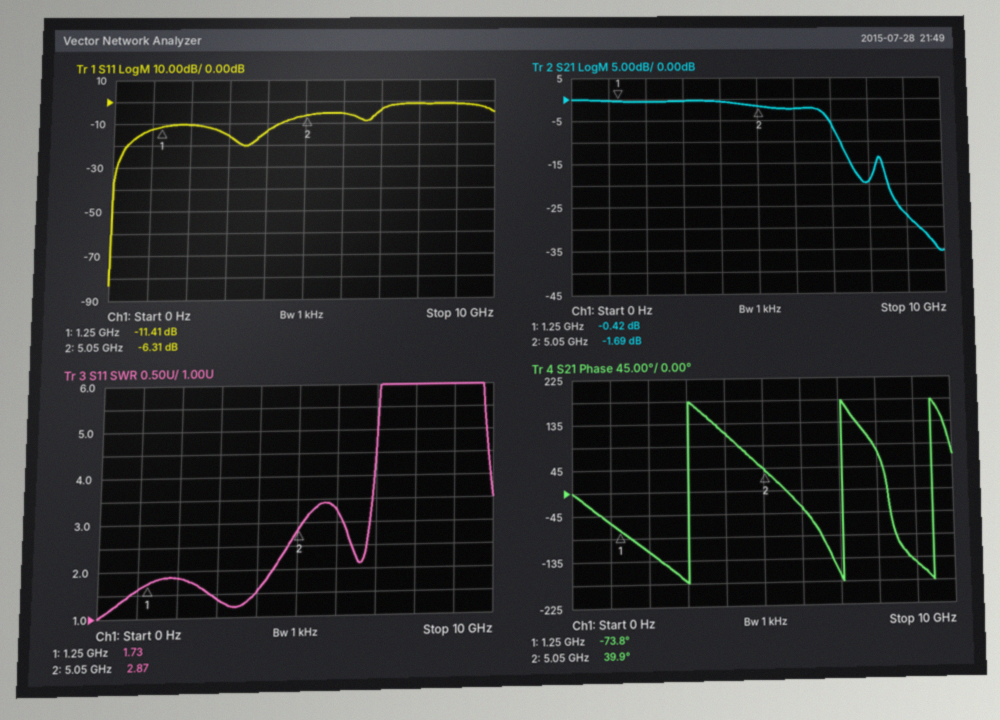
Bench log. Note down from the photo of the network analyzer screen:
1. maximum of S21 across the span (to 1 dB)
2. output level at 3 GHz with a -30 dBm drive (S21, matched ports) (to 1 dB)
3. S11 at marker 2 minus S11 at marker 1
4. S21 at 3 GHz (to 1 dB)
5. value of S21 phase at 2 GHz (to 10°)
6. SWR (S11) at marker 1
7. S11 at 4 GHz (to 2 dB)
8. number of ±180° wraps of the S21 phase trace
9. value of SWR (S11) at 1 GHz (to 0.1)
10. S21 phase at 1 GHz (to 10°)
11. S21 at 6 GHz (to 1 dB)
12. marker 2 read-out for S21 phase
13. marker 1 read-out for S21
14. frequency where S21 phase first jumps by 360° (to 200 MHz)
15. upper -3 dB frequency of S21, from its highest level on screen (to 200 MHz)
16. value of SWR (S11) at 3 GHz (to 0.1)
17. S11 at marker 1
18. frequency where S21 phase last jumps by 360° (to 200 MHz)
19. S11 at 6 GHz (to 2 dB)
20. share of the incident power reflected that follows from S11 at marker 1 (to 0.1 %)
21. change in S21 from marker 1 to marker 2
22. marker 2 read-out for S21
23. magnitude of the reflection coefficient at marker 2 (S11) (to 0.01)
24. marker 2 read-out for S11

0 dB
-30 dBm
5.10 dB
0 dB
-120°
1.73
-14 dB
3
1.6
-60°
-2 dB
39.9°
-0.42 dB
3.0 GHz
6.8 GHz
1.4
-11.41 dB
9.4 GHz
-6 dB
7.2 %
-1.27 dB
-1.69 dB
0.48
-6.31 dB
